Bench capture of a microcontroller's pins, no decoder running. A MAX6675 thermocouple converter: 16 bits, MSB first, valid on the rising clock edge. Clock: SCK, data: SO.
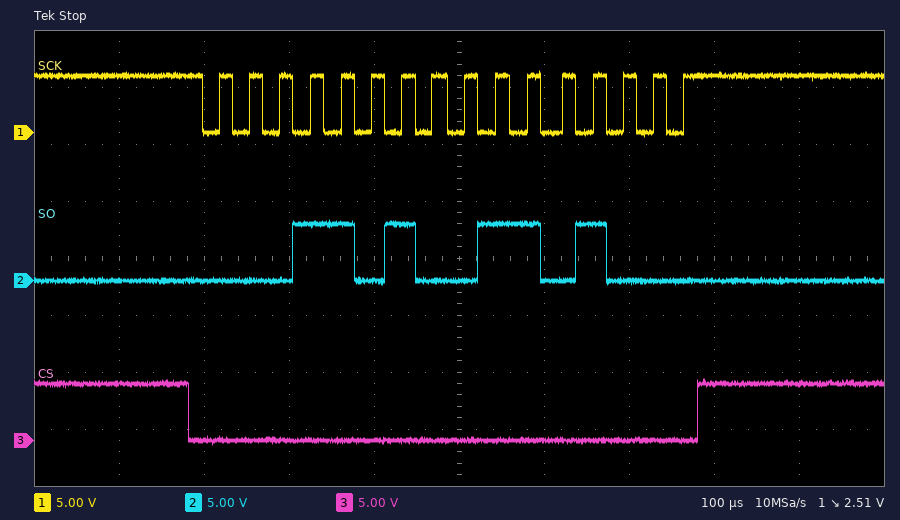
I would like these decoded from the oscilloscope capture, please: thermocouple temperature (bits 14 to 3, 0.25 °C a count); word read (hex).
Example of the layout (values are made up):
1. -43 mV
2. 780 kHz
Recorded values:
1. 211.25 °C
2. 0x1A68
